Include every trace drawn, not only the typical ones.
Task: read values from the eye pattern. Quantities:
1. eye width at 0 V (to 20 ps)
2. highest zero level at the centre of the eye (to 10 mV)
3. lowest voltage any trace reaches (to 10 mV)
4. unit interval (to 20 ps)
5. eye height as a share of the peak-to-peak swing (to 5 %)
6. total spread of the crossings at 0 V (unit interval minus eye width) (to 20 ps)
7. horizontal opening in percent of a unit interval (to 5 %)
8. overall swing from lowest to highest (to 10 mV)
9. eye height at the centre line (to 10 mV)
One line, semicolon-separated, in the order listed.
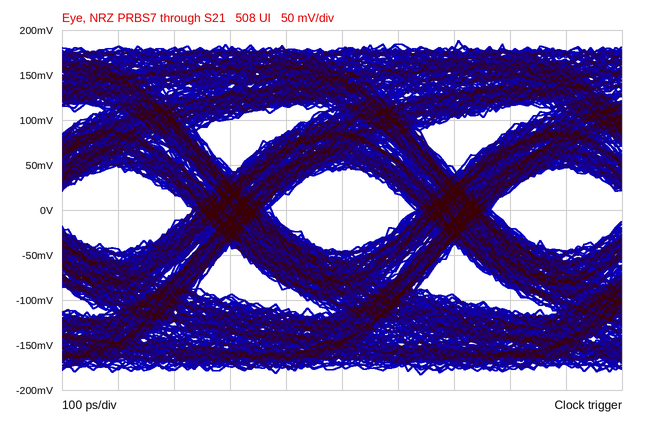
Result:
260 ps; -50 mV; -180 mV; 400 ps; 25 %; 140 ps; 65 %; 370 mV; 90 mV
